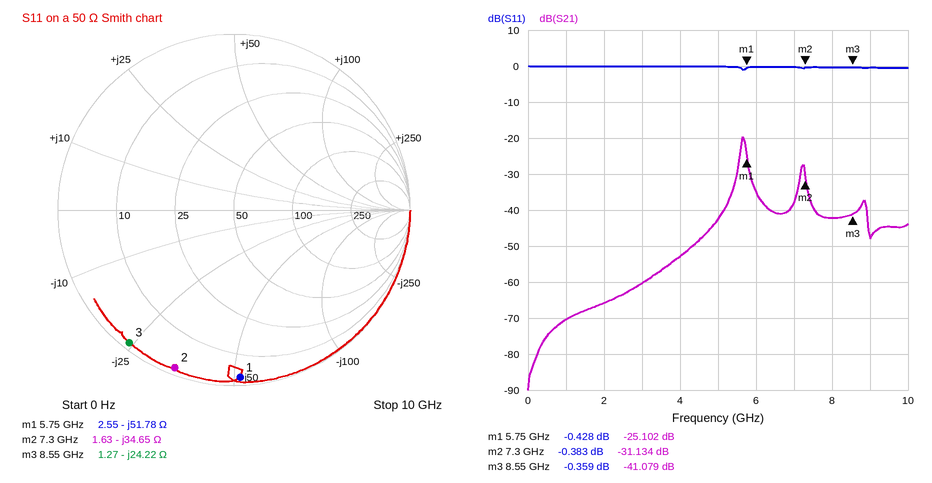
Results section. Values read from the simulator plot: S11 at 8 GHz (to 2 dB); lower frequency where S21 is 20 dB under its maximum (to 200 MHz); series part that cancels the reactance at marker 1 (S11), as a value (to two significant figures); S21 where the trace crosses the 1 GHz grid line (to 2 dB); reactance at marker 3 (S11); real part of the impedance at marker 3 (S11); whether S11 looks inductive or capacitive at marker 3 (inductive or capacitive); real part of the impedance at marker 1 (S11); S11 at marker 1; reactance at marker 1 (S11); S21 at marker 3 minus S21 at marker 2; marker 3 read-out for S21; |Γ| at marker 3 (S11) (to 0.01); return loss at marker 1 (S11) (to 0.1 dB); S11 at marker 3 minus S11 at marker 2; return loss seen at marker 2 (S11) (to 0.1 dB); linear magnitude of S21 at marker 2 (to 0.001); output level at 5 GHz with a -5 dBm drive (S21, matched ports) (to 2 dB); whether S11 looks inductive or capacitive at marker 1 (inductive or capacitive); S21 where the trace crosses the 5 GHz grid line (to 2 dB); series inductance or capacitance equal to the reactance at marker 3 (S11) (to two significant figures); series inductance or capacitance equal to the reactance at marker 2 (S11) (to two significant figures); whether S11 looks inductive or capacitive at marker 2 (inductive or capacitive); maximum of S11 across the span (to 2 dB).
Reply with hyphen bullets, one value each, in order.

- 0 dB
- 5.2 GHz
- 1.4 nH
- -70 dB
- -24.22 Ω
- 1.27 Ω
- capacitive
- 2.55 Ω
- -0.428 dB
- -51.78 Ω
- -9.945 dB
- -41.079 dB
- 0.96
- 0.4 dB
- 0.024 dB
- 0.4 dB
- 0.028
- -48 dBm
- capacitive
- -42 dB
- 770 fF
- 630 fF
- capacitive
- 0 dB
